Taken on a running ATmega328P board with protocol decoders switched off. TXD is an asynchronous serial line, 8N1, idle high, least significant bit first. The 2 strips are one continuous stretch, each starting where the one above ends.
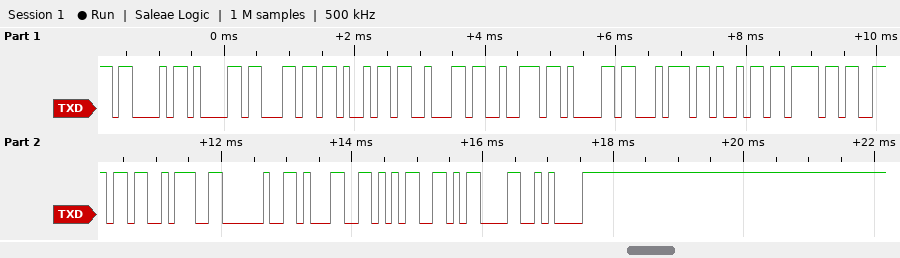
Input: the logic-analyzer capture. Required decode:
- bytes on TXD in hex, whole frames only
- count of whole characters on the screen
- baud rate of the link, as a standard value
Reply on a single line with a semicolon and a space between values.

0x43 0x61 0x6C 0x69 0x62 0x72 0x61 0x74 0x69 0x6F 0x6E 0x3A 0x20 0x31 0x35 0x0D 0x0A; 17; 9600 baud
